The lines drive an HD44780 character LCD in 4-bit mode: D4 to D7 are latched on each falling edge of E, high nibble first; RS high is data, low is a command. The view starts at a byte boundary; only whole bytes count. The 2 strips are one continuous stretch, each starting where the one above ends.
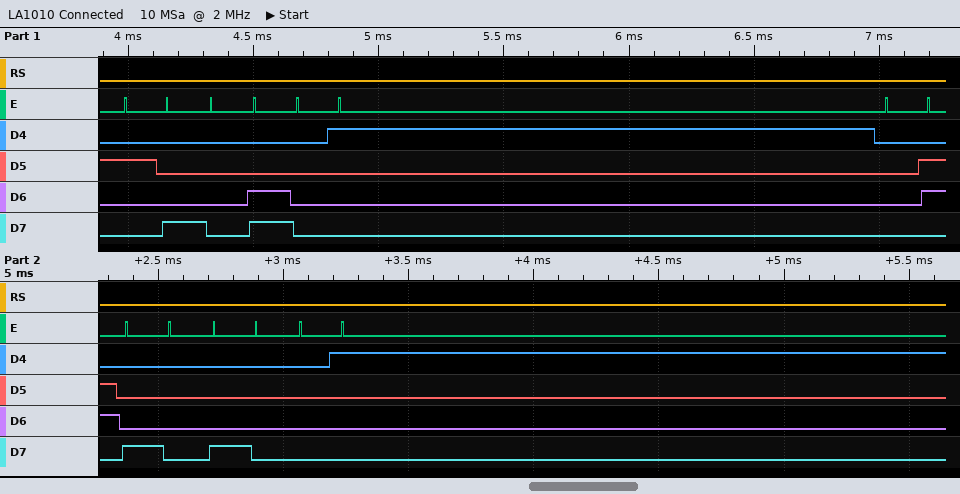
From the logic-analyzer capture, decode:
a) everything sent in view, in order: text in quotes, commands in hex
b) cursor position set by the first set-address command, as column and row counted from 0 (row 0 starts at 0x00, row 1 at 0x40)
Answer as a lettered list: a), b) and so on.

a) 0x28 0x0C 0x01 0x06 0x80 0x80 0x01
b) column 0, row 0
